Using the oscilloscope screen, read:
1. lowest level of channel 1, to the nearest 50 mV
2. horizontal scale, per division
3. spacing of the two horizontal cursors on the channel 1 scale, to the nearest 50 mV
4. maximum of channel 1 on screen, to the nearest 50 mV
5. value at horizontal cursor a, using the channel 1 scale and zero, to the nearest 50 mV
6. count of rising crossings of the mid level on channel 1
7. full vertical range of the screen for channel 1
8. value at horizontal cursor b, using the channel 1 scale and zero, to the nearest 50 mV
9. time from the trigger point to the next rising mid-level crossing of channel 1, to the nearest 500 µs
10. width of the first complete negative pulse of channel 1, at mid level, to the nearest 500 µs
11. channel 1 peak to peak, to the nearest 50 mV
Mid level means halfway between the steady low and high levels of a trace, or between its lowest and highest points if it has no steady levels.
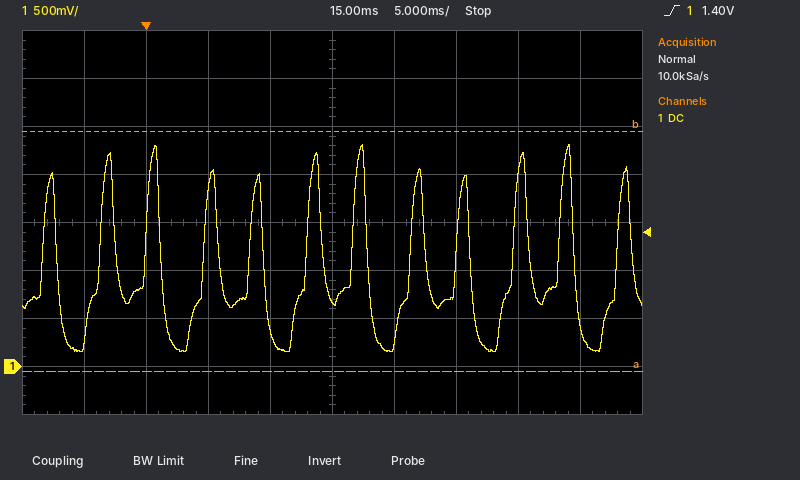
150 mV
5 ms
2.50 V
2.30 V
-50 mV
12
4 V
2.45 V
4.5 ms
3.5 ms
2.15 V
